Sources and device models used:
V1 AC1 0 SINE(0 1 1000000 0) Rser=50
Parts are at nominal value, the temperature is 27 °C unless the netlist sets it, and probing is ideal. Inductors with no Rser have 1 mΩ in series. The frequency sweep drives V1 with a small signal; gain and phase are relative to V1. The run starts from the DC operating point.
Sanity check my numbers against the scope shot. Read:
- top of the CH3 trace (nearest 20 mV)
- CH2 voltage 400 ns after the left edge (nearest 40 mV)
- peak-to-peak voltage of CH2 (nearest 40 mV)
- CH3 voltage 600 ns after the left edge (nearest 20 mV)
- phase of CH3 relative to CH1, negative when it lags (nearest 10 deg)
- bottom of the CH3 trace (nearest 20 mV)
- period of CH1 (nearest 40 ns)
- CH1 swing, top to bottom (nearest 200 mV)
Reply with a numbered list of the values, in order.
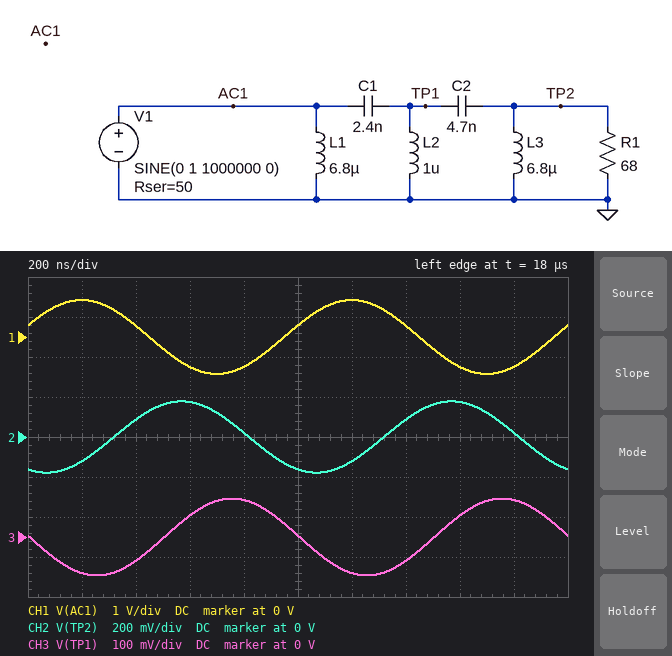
1. 100 mV
2. 80 mV
3. 360 mV
4. 60 mV
5. 160 deg
6. -100 mV
7. 1.00 µs
8. 1.8 V
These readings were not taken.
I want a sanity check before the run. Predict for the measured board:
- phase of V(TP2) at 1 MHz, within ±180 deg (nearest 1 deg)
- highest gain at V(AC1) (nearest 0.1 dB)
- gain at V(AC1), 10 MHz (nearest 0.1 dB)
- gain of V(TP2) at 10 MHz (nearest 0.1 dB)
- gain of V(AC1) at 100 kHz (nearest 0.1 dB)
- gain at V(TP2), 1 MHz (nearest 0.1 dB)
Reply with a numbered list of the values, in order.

1. -115 deg
2. -0.3 dB
3. -6.8 dB
4. -5.7 dB
5. -21.3 dB
6. -15.0 dB
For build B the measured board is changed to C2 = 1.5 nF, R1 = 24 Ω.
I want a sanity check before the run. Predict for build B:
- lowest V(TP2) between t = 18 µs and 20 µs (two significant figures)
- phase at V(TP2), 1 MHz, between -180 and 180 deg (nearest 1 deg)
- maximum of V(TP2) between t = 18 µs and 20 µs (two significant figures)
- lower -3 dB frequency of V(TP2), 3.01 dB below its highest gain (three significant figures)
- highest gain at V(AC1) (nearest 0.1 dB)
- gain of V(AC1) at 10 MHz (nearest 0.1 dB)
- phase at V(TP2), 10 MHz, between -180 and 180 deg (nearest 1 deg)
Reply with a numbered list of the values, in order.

1. -23 mV
2. -54 deg
3. 23 mV
4. 2.69 MHz
5. 0 dB
6. -8.8 dB
7. 34 deg
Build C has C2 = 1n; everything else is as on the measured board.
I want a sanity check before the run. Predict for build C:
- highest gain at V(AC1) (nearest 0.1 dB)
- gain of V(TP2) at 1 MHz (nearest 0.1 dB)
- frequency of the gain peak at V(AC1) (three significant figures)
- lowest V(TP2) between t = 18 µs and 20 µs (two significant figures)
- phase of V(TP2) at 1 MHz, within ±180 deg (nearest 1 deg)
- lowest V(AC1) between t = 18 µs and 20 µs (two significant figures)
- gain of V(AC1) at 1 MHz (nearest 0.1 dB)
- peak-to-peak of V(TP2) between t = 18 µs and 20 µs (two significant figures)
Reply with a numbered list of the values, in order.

1. 0 dB
2. -30.7 dB
3. 1.15 MHz
4. -29 mV
5. -23 deg
6. -950 mV
7. -0.5 dB
8. 58 mV
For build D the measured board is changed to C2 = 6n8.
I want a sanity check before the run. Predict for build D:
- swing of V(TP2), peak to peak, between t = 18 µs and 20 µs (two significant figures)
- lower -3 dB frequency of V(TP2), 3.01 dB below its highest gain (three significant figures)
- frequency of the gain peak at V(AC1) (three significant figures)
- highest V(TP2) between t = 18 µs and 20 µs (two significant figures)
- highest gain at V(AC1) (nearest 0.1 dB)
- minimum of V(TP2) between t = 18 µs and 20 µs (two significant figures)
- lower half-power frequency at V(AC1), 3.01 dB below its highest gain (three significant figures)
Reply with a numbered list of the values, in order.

1. 290 mV
2. 4.74 MHz
3. 1.16 MHz
4. 150 mV
5. -0.2 dB
6. -150 mV
7. 724 kHz
